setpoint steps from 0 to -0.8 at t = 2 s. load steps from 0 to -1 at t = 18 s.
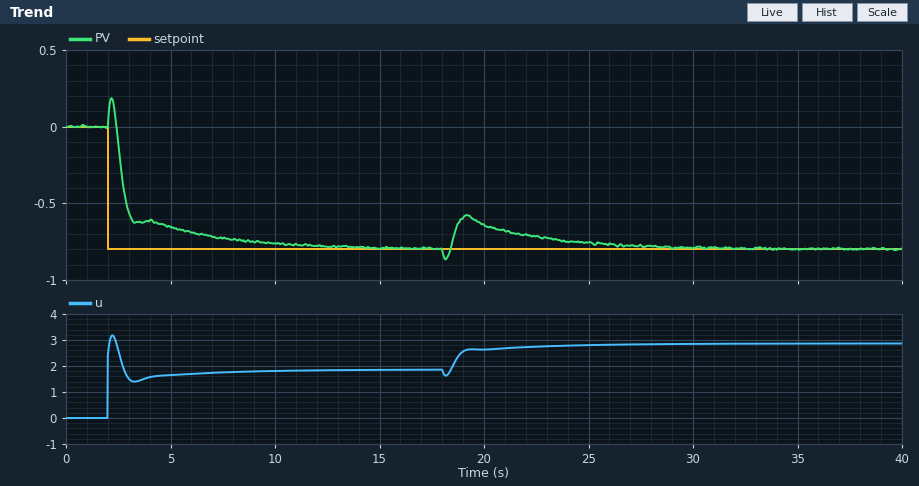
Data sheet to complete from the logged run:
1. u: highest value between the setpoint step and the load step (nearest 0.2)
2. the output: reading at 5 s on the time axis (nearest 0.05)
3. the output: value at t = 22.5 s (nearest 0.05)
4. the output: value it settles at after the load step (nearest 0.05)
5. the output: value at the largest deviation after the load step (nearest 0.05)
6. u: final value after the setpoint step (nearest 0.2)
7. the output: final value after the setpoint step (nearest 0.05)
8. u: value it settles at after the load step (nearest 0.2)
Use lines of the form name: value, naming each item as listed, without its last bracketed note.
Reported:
u: highest value between the setpoint step and the load step: 3.2
the output: reading at 5 s on the time axis: -0.65
the output: value at t = 22.5 s: -0.70
the output: value it settles at after the load step: -0.80
the output: value at the largest deviation after the load step: -0.60
u: final value after the setpoint step: 1.8
the output: final value after the setpoint step: -0.80
u: value it settles at after the load step: 2.8
